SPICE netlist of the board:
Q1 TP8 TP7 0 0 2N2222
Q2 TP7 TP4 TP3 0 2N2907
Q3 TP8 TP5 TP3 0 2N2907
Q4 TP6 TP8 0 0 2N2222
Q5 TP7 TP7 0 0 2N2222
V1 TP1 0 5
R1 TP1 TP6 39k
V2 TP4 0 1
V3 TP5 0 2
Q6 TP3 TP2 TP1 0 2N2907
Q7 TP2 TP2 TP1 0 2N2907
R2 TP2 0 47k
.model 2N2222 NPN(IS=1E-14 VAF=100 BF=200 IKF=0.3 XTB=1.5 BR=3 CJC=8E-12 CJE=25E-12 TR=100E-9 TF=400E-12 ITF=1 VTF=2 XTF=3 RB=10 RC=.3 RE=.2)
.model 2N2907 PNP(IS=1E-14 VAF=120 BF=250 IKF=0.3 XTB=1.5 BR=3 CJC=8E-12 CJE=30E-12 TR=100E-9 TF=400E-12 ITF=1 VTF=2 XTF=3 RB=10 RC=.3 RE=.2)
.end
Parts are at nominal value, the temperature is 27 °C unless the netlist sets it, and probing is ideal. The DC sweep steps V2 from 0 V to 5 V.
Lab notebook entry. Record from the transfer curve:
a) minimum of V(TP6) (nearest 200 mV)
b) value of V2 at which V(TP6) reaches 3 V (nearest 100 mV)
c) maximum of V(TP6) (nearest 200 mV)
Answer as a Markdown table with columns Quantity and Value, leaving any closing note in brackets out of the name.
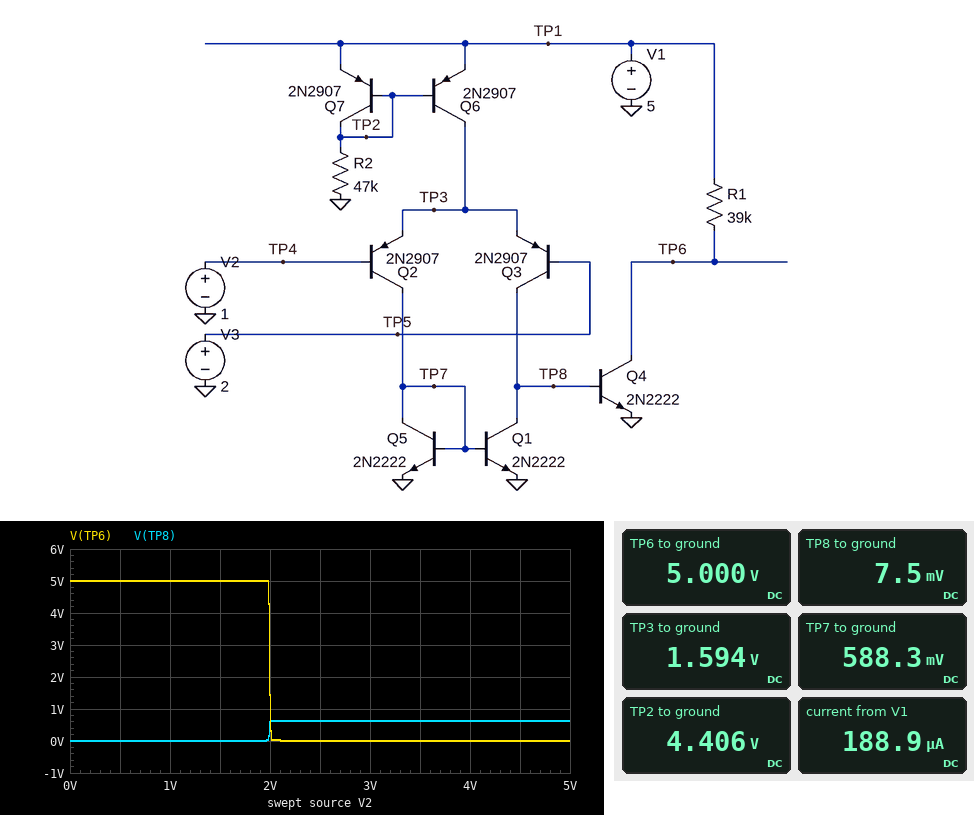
| Quantity | Value |
|---|---|
| minimum of V(TP6) | 0 V |
| value of V2 at which V(TP6) reaches 3 V | 2.0 V |
| maximum of V(TP6) | 5.0 V |
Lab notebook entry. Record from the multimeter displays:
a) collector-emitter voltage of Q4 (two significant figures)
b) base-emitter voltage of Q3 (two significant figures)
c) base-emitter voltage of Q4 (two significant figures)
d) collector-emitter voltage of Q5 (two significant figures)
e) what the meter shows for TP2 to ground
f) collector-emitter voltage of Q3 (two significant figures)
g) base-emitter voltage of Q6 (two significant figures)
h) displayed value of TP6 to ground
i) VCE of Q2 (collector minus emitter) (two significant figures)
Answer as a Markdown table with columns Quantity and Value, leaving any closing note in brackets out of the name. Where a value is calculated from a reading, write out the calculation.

| Quantity | Value |
|---|---|
| collector-emitter voltage of Q4 | 5 V = 5.0 V |
| base-emitter voltage of Q3 | 2 V - 1.594 V = 410 mV |
| base-emitter voltage of Q4 | 7.5 mV = 7.5 mV |
| collector-emitter voltage of Q5 | 588.3 mV = 590 mV |
| what the meter shows for TP2 to ground | 4.406 V |
| collector-emitter voltage of Q3 | 7.5 mV - 1.594 V = -1.6 V |
| base-emitter voltage of Q6 | 4.406 V - 5 V = -590 mV |
| displayed value of TP6 to ground | 5.000 V |
| VCE of Q2 (collector minus emitter) | 588.3 mV - 1.594 V = -1.0 V |
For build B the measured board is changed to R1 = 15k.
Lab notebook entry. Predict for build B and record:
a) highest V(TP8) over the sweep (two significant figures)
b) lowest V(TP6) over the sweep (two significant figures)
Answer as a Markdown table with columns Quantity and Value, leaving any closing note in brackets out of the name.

| Quantity | Value |
|---|---|
| highest V(TP8) over the sweep | 650 mV |
| lowest V(TP6) over the sweep | 25 mV |
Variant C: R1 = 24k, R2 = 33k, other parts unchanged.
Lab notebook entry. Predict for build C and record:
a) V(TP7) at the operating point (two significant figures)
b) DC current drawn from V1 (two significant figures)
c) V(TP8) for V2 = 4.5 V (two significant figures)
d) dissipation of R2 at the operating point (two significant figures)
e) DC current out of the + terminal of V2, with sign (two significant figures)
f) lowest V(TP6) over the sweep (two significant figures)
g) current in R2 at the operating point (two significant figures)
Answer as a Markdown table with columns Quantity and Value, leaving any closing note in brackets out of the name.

| Quantity | Value |
|---|---|
| V(TP7) at the operating point | 600 mV |
| DC current drawn from V1 | 270 µA |
| V(TP8) for V2 = 4.5 V | 650 mV |
| dissipation of R2 at the operating point | 590 µW |
| DC current out of the + terminal of V2, with sign | -540 nA |
| lowest V(TP6) over the sweep | 16 mV |
| current in R2 at the operating point | 130 µA |
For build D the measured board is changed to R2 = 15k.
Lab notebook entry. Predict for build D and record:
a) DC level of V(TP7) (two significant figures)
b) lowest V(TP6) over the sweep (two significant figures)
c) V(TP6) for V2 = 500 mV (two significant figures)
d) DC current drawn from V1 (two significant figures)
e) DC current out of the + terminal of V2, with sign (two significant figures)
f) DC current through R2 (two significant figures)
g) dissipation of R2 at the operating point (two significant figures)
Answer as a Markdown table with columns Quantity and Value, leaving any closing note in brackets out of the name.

| Quantity | Value |
|---|---|
| DC level of V(TP7) | 620 mV |
| lowest V(TP6) over the sweep | 10 mV |
| V(TP6) for V2 = 500 mV | 5.0 V |
| DC current drawn from V1 | 590 µA |
| DC current out of the + terminal of V2, with sign | -1.2 µA |
| DC current through R2 | 290 µA |
| dissipation of R2 at the operating point | 1.3 mW |
